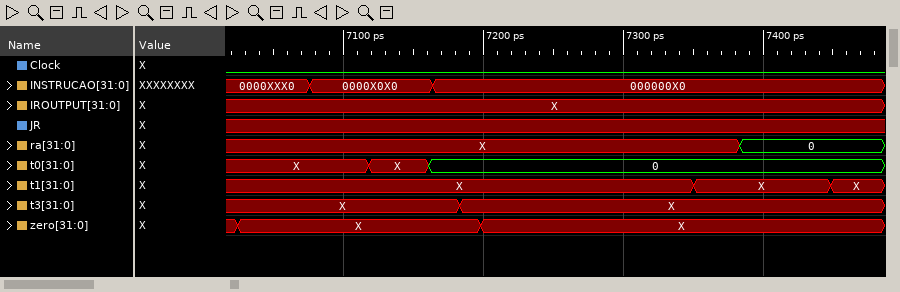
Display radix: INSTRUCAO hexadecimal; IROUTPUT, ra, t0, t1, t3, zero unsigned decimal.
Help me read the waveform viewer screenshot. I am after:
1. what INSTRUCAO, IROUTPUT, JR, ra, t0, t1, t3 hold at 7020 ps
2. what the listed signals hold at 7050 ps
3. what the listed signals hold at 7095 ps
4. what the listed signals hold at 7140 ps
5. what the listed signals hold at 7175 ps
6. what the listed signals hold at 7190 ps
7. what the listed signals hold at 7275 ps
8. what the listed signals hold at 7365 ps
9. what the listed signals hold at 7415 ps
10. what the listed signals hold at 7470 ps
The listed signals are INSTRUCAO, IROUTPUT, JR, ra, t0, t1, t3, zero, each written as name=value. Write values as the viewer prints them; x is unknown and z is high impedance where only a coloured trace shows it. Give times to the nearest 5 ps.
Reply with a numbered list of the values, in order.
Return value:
1. INSTRUCAO=0000XXX0, IROUTPUT=X, JR=x, ra=X, t0=X, t1=X, t3=X
2. INSTRUCAO=0000XXX0, IROUTPUT=X, JR=x, ra=X, t0=X, t1=X, t3=X, zero=X
3. INSTRUCAO=0000X0X0, IROUTPUT=X, JR=x, ra=X, t0=X, t1=X, t3=X, zero=X
4. INSTRUCAO=0000X0X0, IROUTPUT=X, JR=x, ra=X, t0=X, t1=X, t3=X, zero=X
5. INSTRUCAO=000000X0, IROUTPUT=X, JR=x, ra=X, t0=0, t1=X, t3=X, zero=X
6. INSTRUCAO=000000X0, IROUTPUT=X, JR=x, ra=X, t0=0, t1=X, t3=X, zero=X
7. INSTRUCAO=000000X0, IROUTPUT=X, JR=x, ra=X, t0=0, t1=X, t3=X, zero=X
8. INSTRUCAO=000000X0, IROUTPUT=X, JR=x, ra=X, t0=0, t1=X, t3=X, zero=X
9. INSTRUCAO=000000X0, IROUTPUT=X, JR=x, ra=0, t0=0, t1=X, t3=X, zero=X
10. INSTRUCAO=000000X0, IROUTPUT=X, JR=x, ra=0, t0=0, t1=X, t3=X, zero=X
